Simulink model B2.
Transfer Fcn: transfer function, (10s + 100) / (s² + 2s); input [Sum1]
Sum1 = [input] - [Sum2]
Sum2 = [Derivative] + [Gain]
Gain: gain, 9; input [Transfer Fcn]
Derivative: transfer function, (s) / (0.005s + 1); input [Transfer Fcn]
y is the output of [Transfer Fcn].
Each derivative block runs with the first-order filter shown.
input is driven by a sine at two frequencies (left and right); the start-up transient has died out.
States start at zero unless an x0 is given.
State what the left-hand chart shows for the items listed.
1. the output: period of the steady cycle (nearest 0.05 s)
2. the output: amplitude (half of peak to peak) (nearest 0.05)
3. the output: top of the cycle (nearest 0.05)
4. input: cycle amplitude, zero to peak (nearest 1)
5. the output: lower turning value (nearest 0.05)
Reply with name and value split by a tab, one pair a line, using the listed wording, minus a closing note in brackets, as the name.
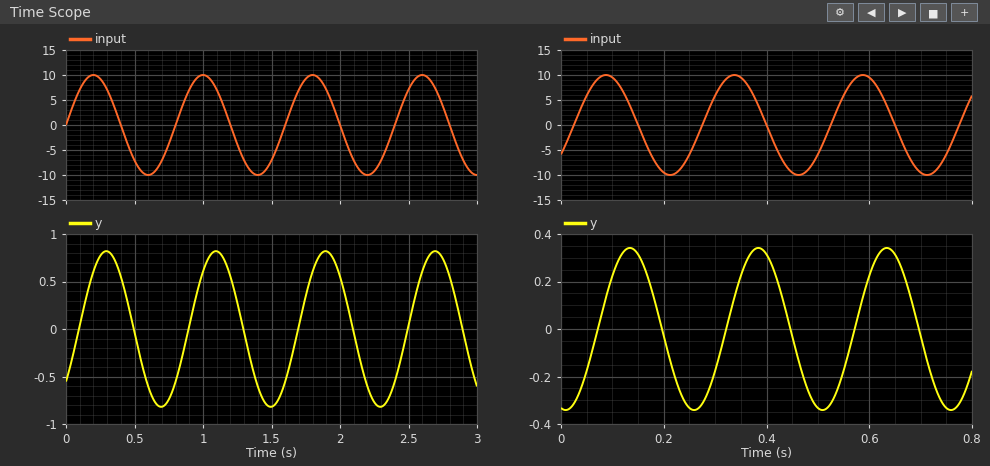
the output: period of the steady cycle	0.80 s
the output: amplitude (half of peak to peak)	0.80
the output: top of the cycle	0.80
input: cycle amplitude, zero to peak	10
the output: lower turning value	-0.80
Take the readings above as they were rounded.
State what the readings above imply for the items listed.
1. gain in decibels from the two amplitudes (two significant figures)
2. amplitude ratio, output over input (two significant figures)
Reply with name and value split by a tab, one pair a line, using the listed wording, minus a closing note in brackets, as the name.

gain in decibels from the two amplitudes	-22 dB
amplitude ratio, output over input	0.080
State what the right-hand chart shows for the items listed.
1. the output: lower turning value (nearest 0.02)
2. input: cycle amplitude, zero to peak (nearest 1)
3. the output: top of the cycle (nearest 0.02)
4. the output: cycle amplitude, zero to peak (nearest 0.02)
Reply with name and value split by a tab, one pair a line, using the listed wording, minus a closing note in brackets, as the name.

the output: lower turning value	-0.34
input: cycle amplitude, zero to peak	10
the output: top of the cycle	0.34
the output: cycle amplitude, zero to peak	0.34
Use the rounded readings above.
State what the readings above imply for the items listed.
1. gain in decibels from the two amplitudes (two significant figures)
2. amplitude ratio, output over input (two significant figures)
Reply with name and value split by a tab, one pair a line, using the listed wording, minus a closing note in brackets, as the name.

gain in decibels from the two amplitudes	-29 dB
amplitude ratio, output over input	0.034
